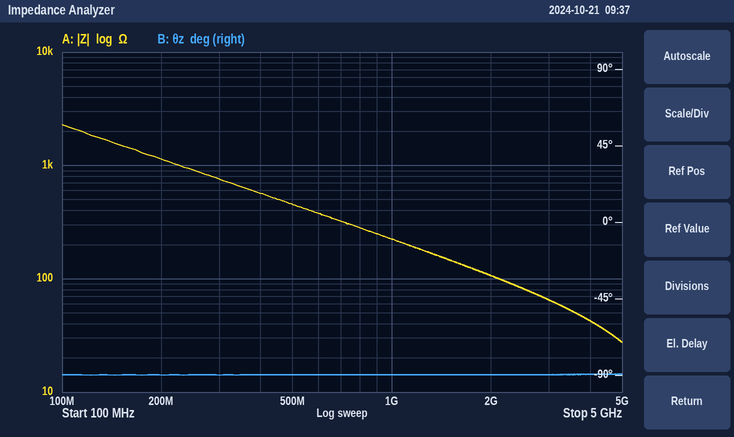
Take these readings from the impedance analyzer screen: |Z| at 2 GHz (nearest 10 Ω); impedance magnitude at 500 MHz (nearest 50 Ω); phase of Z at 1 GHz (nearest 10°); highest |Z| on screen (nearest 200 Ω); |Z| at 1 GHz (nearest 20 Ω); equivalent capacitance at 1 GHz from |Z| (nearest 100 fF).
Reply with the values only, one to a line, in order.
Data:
110 Ω
450 Ω
-90°
2.2 kΩ
220 Ω
700 fF
